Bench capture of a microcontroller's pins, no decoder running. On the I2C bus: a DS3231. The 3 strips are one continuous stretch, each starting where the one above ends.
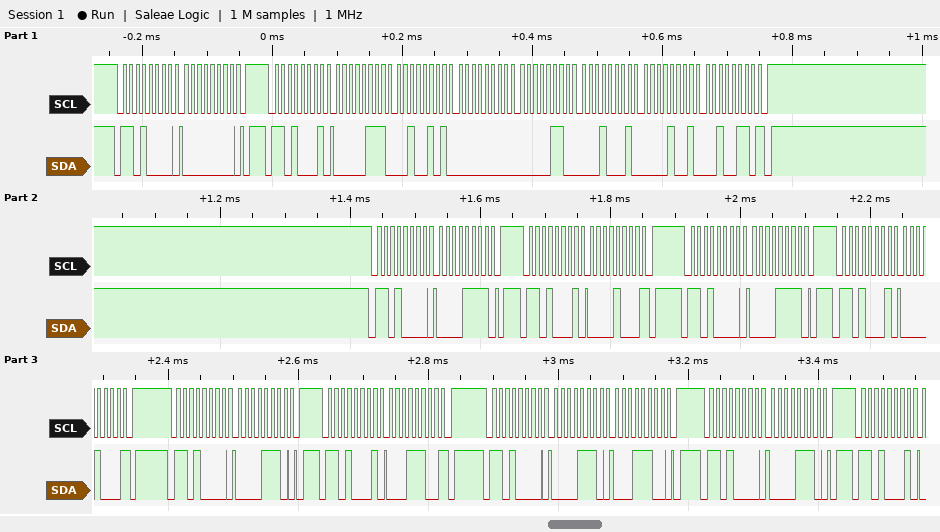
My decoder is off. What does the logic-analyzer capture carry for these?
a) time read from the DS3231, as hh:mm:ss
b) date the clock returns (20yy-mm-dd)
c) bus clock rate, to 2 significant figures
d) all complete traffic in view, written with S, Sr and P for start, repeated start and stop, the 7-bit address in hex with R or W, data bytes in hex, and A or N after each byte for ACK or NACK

00:25:07
2026-09-11
100 kHz
S 68W A 00 A P S 68R A 07 A 25 A 00 A 06 A 11 A 09 A 26 N P S 68W A 0F A P S 68R A 08 N P S 68W A 0F A P S 68R A 08 N P S 68W A 0E A P S 68R A 1C N P S 68W A 0E A 1C A P S 68W A 0E A P S 68R A
